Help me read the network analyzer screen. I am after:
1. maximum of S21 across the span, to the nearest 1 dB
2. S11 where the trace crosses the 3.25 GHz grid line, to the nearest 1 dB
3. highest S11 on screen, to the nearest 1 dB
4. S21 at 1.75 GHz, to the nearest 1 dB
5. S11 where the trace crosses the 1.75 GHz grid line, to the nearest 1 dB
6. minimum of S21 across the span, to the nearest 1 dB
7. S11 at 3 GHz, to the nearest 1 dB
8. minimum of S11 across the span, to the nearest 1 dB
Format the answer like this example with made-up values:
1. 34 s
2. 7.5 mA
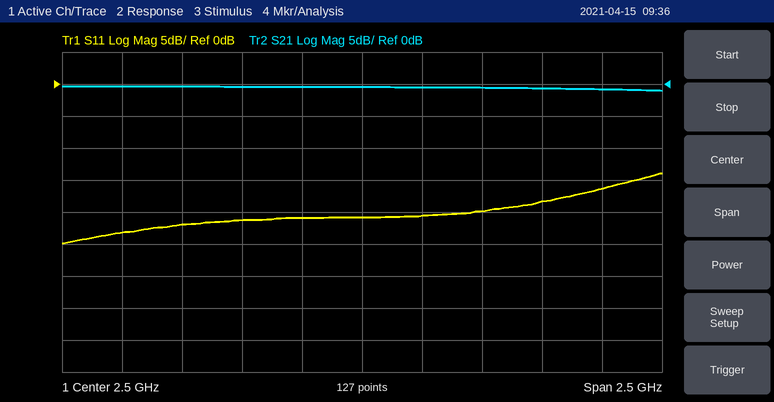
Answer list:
1. 0 dB
2. -18 dB
3. -14 dB
4. 0 dB
5. -22 dB
6. -1 dB
7. -20 dB
8. -25 dB
